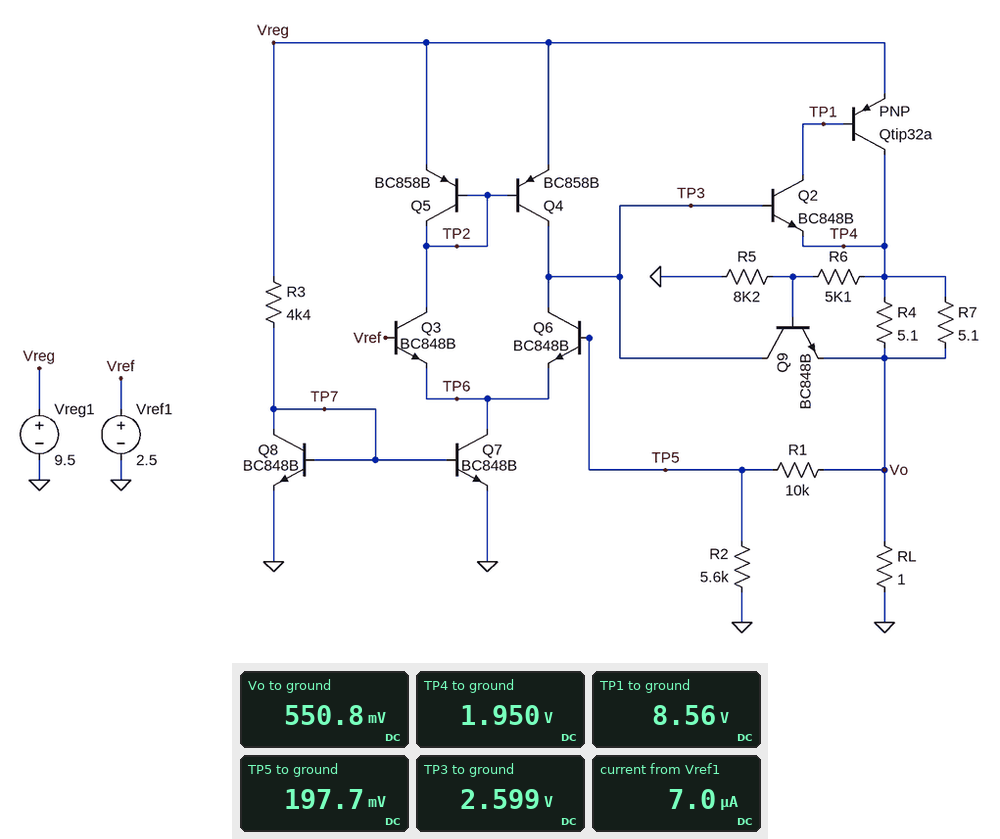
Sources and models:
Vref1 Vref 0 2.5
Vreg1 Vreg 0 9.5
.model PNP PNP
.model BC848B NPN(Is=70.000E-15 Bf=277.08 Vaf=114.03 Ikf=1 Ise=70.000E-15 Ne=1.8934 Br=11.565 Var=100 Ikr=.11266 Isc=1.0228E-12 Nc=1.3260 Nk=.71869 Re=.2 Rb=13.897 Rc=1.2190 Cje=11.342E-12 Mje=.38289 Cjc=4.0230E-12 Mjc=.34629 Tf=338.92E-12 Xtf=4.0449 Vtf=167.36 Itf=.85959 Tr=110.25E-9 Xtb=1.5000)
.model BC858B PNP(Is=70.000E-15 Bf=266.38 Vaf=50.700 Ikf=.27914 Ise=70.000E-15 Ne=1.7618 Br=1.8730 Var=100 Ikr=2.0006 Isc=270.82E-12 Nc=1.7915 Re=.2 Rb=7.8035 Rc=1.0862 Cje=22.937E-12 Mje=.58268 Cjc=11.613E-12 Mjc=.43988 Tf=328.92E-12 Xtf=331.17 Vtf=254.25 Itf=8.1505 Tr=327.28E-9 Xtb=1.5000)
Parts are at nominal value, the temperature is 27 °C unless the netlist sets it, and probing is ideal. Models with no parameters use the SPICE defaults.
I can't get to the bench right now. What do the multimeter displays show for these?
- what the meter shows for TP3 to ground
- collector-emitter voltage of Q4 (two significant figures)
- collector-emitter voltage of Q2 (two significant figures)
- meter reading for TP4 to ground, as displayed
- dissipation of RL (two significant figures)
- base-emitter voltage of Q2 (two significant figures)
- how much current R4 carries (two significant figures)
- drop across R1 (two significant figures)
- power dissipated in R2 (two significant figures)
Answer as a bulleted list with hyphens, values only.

- 2.599 V
- -6.9 V
- 6.6 V
- 1.950 V
- 300 mW
- 650 mV
- 270 mA
- 350 mV
- 7.0 µW
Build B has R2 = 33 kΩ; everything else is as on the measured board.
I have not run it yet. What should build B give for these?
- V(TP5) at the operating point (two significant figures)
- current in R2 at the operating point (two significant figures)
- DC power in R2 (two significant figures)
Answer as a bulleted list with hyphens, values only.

- 420 mV
- 13 µA
- 5.4 µW
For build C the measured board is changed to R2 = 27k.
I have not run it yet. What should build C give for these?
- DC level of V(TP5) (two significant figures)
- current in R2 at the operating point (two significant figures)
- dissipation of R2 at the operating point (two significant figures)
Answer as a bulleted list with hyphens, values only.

- 400 mV
- 15 µA
- 6.0 µW
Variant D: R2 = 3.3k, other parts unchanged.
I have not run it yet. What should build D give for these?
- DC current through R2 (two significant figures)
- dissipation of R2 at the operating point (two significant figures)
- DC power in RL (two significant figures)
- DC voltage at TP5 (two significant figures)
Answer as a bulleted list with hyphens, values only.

- 41 µA
- 5.7 µW
- 300 mW
- 140 mV
